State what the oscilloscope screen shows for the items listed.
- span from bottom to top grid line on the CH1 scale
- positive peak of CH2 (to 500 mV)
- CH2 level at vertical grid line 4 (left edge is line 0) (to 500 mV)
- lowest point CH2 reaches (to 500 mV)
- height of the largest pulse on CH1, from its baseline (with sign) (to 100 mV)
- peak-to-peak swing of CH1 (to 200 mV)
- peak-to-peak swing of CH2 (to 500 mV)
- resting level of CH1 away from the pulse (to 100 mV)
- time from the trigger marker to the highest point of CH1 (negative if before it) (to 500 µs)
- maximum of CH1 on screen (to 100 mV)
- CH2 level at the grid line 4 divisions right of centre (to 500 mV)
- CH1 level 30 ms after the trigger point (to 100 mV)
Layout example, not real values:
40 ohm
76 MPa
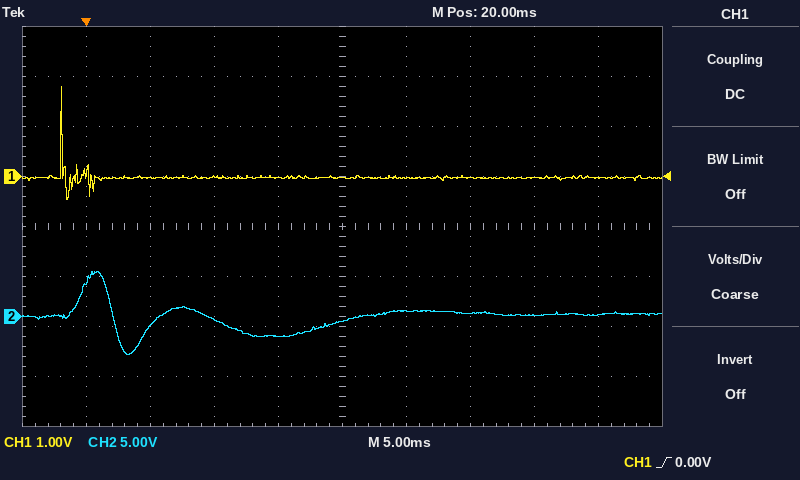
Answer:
8 V
4.5 V
-2.0 V
-4.0 V
+1.8 V
2.2 V
8.5 V
0.0 V
-2.0 ms
1.8 V
0.0 V
0.0 V
